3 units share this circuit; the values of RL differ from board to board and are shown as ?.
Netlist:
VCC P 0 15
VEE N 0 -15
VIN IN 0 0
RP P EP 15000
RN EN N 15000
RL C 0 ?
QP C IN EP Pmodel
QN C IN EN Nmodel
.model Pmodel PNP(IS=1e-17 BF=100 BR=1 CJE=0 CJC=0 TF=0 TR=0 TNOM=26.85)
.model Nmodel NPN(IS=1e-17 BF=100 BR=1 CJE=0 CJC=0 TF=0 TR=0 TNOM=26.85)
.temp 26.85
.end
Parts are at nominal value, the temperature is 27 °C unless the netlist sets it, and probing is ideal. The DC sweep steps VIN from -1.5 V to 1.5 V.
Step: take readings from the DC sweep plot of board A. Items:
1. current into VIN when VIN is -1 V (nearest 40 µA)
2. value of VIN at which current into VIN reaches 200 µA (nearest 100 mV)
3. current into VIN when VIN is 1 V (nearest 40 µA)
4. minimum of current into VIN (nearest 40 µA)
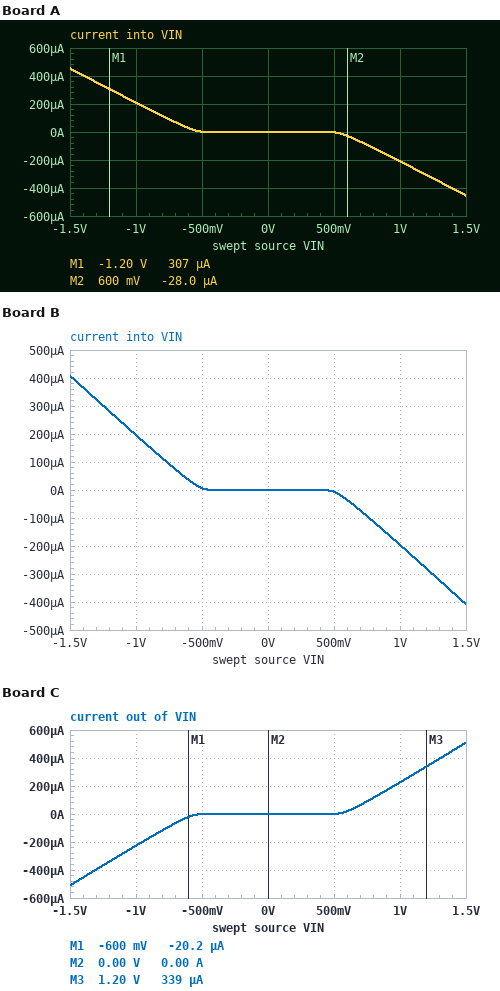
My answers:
200 µA
-1.0 V
-200 µA
-440 µA
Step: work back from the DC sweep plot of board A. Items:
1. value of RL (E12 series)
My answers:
2.7 kΩ
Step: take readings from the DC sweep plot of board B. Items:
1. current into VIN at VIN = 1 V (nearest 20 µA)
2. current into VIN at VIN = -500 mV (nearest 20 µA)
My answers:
-200 µA
0 A
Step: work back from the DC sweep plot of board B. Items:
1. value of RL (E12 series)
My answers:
3.3 kΩ
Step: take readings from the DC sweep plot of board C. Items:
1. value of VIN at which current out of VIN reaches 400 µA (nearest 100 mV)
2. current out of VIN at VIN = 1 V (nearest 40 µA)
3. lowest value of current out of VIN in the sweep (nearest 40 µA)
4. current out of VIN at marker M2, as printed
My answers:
1.3 V
240 µA
-520 µA
0.00 A
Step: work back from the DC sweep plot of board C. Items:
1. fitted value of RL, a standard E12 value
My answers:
2.2 kΩ
